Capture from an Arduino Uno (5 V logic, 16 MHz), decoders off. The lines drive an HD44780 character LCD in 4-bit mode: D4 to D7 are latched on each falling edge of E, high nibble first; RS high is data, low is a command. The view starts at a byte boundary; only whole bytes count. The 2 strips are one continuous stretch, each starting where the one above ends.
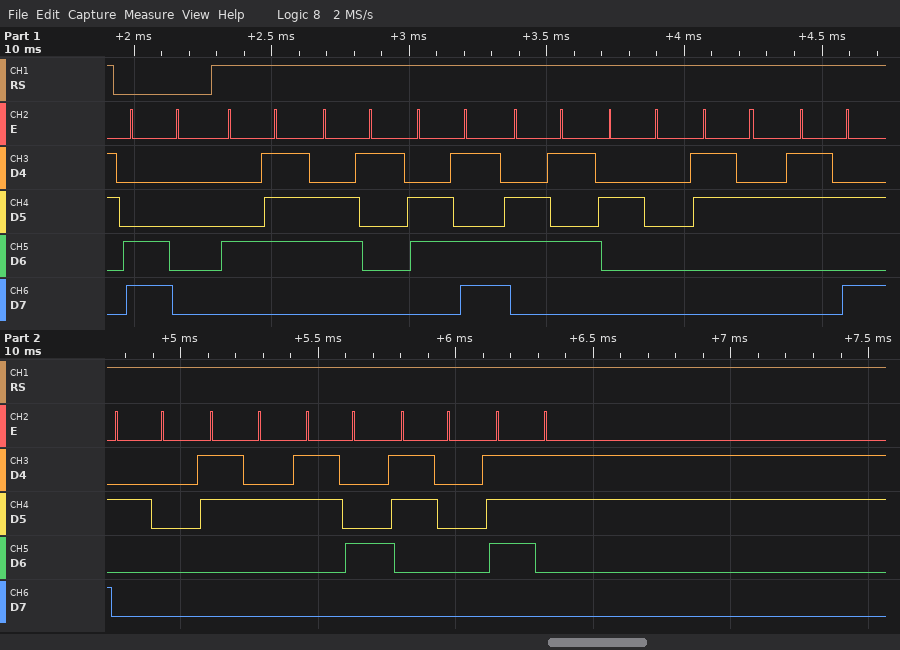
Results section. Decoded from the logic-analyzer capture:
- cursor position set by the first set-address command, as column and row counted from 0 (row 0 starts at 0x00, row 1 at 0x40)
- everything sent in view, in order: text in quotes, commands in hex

column 0, row 1
0xC0 "Game 2: 240s"
